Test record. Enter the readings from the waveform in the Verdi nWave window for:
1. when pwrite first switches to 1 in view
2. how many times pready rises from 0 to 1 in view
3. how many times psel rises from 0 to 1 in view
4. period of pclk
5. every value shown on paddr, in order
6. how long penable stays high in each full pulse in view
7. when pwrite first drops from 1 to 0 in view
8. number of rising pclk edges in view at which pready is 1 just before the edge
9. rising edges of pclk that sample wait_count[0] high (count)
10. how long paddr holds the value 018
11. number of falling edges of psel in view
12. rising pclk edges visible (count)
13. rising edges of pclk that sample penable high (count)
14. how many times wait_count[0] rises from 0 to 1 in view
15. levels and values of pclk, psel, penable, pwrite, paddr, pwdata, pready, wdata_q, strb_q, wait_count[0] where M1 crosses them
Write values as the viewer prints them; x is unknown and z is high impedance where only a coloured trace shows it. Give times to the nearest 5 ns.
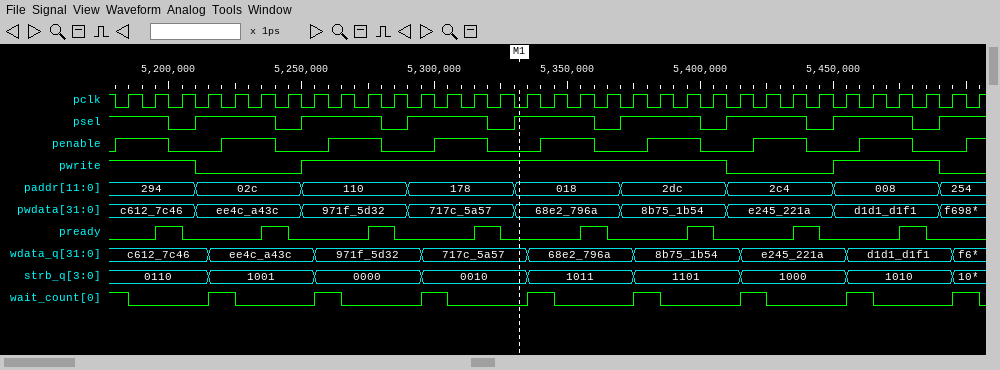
5250 ns
8
8
10 ns
294, 02c, 110, 178, 018, 2dc, 2c4, 008, 254
20 ns, 20 ns, 20 ns, 20 ns, 20 ns, 20 ns, 20 ns, 20 ns
5210 ns
8
9
40 ns
8
33
17
8
pclk=0, psel=1, penable=0, pwrite=1, paddr=018, pwdata=68e2_796a, pready=0, wdata_q=717c_5a57, strb_q=0010, wait_count[0]=0
